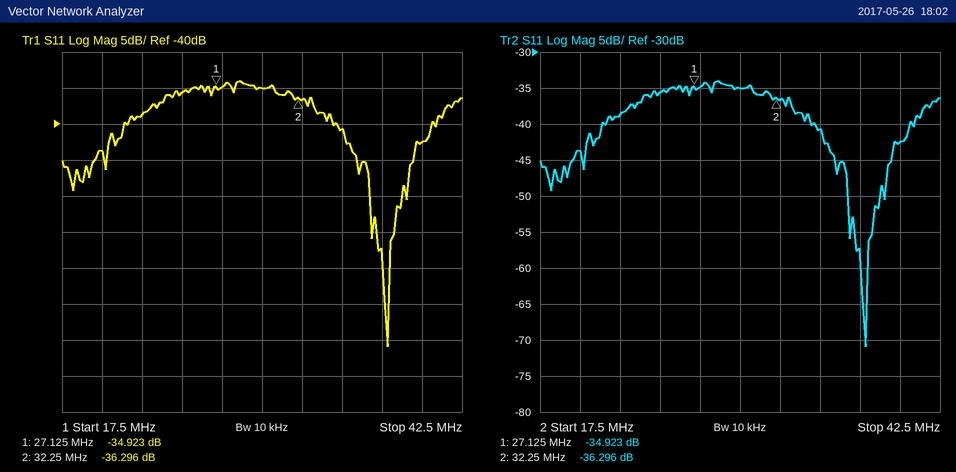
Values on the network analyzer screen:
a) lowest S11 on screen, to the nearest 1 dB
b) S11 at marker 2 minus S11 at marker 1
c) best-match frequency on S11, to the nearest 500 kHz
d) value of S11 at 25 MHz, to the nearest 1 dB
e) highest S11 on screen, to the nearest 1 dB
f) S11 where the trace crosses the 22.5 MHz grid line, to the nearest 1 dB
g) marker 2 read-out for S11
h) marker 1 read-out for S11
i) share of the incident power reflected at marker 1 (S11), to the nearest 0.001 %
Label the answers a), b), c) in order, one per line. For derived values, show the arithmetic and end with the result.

a) -71 dB
b) -36.296 − (-34.923) = -1.373 dB
c) 38.0 MHz
d) -36 dB
e) -34 dB
f) -39 dB
g) -36.296 dB
h) -34.923 dB
i) 10^(-34.923/10) ≈ 0.032 %
